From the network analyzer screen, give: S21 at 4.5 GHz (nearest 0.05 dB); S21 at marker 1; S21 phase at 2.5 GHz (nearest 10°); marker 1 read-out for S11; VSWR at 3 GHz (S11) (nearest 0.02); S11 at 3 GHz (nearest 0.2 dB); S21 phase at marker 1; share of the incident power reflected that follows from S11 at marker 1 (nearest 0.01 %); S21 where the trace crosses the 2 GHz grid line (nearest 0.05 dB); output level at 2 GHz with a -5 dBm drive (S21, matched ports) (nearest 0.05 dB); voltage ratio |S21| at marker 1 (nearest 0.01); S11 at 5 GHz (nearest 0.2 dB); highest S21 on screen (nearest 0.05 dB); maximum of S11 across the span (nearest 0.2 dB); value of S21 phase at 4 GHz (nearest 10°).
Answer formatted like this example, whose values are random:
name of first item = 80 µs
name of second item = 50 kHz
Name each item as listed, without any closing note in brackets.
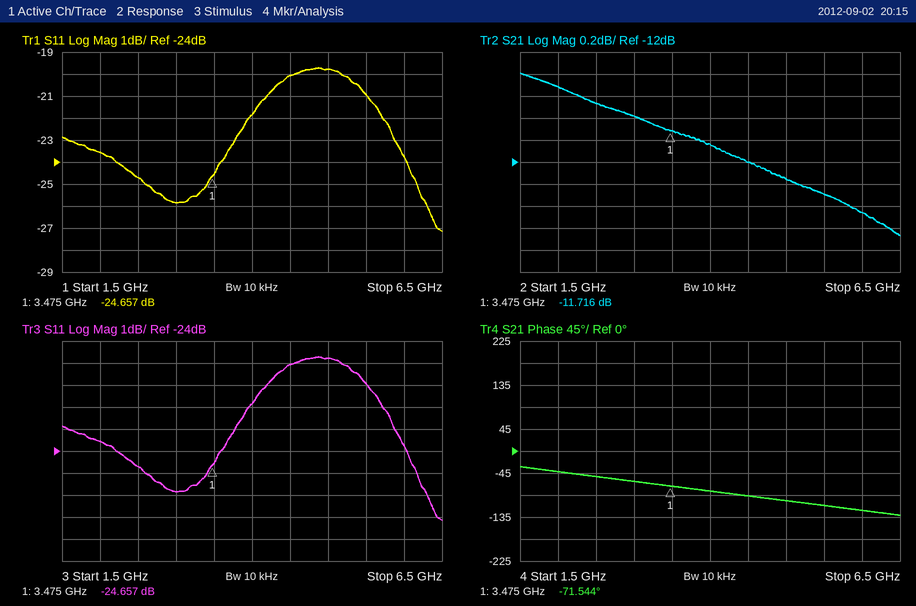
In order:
S21 at 4.5 GHz = -12.00 dB
S21 at marker 1 = -11.716 dB
S21 phase at 2.5 GHz = -50°
marker 1 read-out for S11 = -24.657 dB
VSWR at 3 GHz (S11) = 1.10
S11 at 3 GHz = -25.8 dB
S21 phase at marker 1 = -71.544°
share of the incident power reflected that follows from S11 at marker 1 = 0.34 %
S21 where the trace crosses the 2 GHz grid line = -11.30 dB
output level at 2 GHz with a -5 dBm drive (S21, matched ports) = -16.30 dBm
voltage ratio |S21| at marker 1 = 0.26
S11 at 5 GHz = -19.8 dB
highest S21 on screen = -11.20 dB
maximum of S11 across the span = -19.8 dB
value of S21 phase at 4 GHz = -80°
